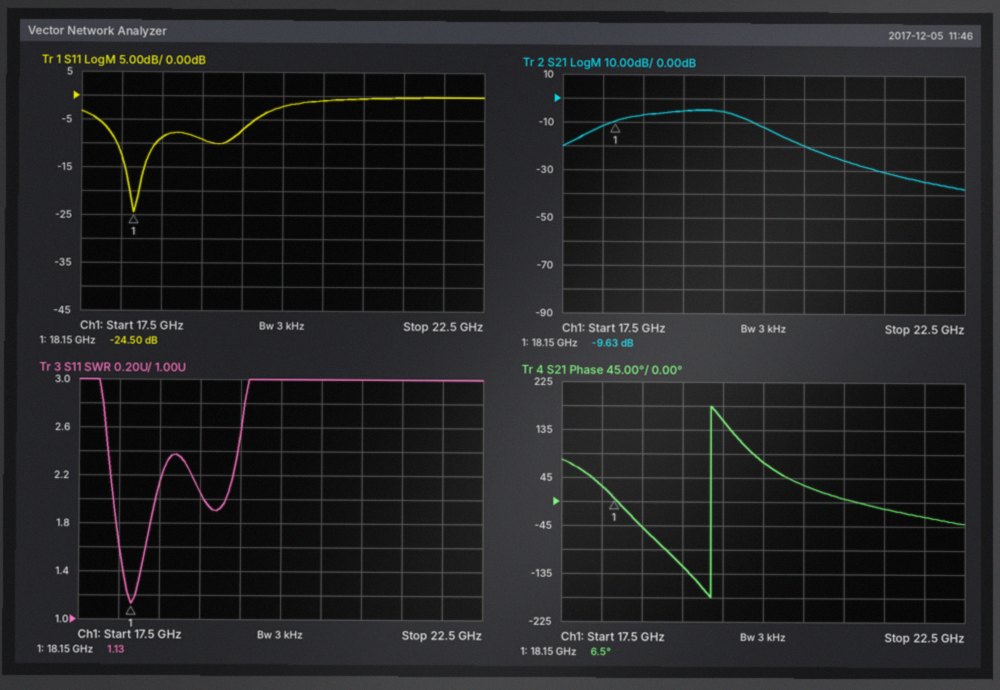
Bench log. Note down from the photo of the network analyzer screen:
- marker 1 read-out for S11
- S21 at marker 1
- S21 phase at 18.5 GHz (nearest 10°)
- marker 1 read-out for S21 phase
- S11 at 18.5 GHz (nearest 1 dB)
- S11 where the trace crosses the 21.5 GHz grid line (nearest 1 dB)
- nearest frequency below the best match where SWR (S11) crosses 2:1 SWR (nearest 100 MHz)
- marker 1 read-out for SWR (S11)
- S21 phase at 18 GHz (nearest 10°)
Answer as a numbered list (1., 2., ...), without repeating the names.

1. -24.50 dB
2. -9.63 dB
3. -50°
4. 6.5°
5. -9 dB
6. 0 dB
7. 17.9 GHz
8. 1.13
9. 30°
